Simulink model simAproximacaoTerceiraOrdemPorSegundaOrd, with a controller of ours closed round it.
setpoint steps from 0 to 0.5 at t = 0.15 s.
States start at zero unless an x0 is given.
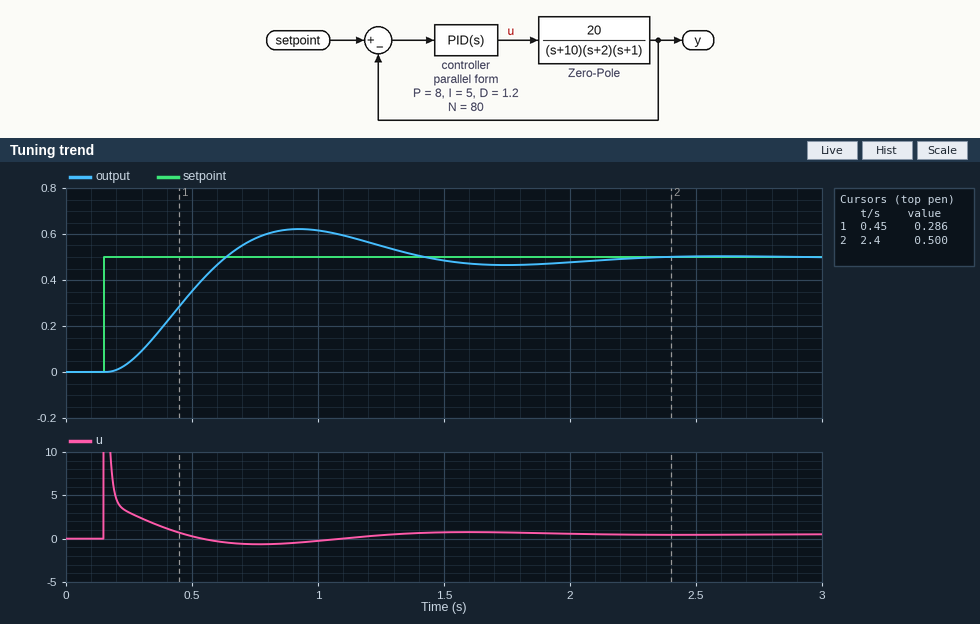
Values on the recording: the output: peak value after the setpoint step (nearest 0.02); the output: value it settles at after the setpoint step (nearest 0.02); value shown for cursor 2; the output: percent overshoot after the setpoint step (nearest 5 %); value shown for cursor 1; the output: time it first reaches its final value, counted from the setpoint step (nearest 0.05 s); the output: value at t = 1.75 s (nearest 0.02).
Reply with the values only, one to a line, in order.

0.62
0.50
0.500
25 %
0.286
0.50 s
0.46
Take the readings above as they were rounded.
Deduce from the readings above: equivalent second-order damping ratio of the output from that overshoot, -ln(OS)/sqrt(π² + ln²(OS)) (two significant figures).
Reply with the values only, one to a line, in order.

0.40
